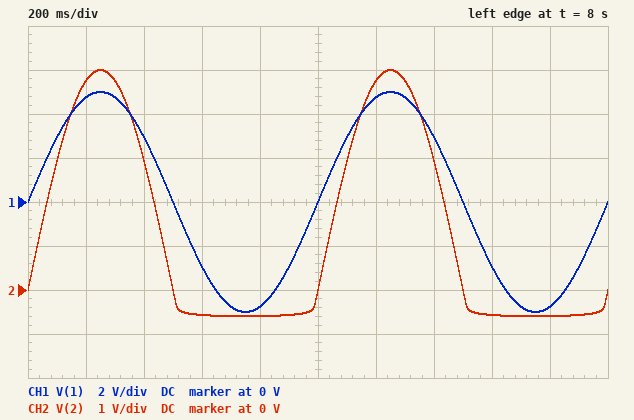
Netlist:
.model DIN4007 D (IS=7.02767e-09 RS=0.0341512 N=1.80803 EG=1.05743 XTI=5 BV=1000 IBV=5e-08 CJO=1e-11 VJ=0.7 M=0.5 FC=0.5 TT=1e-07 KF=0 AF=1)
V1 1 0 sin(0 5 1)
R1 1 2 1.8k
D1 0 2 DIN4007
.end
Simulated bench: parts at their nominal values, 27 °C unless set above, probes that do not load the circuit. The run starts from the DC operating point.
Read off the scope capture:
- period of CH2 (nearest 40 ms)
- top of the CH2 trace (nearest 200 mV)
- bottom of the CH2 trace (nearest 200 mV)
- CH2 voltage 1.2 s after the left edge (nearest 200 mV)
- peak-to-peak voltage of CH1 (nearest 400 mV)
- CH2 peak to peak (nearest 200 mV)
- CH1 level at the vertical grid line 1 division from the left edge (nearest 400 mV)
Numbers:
1.00 s
5.0 V
-600 mV
4.8 V
10.0 V
5.6 V
4.8 V
